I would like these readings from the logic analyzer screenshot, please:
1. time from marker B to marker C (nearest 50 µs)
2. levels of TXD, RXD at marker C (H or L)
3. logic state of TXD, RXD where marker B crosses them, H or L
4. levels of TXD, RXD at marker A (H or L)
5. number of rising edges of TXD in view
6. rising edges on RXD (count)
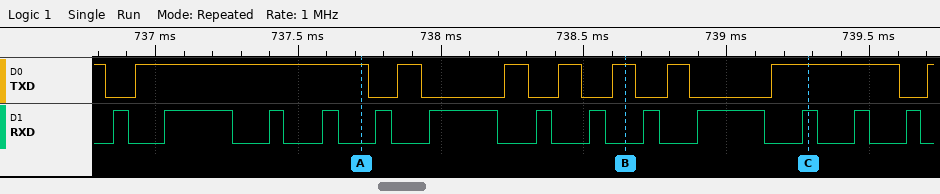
650 µs
TXD=H, RXD=H
TXD=H, RXD=L
TXD=H, RXD=L
8
13
